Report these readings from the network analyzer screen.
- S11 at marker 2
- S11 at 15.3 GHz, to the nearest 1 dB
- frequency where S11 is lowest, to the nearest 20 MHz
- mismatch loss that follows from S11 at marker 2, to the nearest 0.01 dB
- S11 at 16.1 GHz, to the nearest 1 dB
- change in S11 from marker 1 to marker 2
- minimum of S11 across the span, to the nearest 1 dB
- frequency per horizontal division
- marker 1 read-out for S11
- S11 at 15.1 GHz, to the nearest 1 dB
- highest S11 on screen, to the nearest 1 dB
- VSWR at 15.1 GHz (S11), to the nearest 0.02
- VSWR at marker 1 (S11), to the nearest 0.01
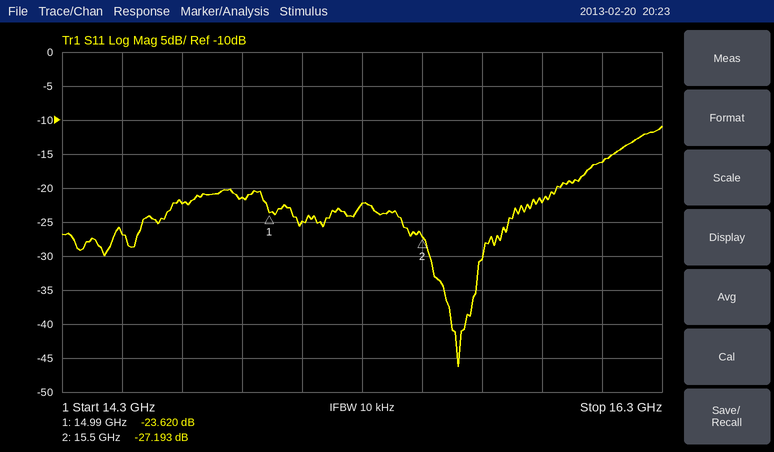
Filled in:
-27.193 dB
-22 dB
15.62 GHz
0.01 dB
-16 dB
-3.573 dB
-46 dB
200 MHz
-23.620 dB
-25 dB
-11 dB
1.12
1.14
